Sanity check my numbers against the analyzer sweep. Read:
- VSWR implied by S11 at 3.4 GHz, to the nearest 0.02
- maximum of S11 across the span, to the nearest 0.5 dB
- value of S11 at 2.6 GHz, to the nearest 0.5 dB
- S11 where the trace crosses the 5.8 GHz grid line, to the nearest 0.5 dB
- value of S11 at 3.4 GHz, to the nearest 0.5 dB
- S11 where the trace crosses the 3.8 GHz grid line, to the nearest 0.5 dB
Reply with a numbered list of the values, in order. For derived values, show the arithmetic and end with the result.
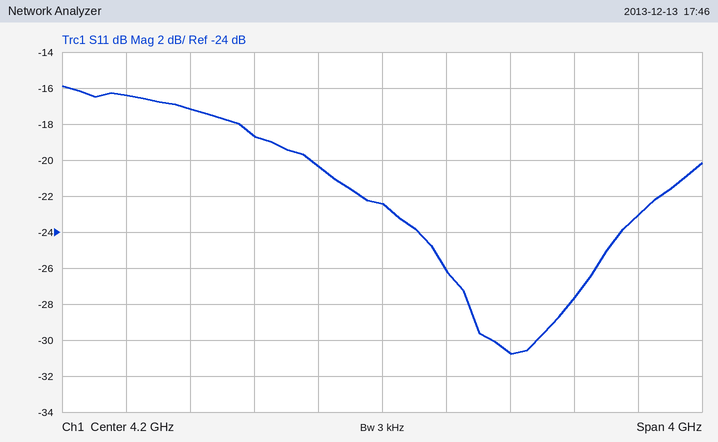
1. |Γ| = 10^(-18.5/20) = 0.1189; VSWR = (1 + 0.1189)/(1 − 0.1189) ≈ 1.27, so 1.26 to the nearest 0.02
2. -16.0 dB
3. -16.5 dB
4. -23.0 dB
5. -18.5 dB
6. -20.5 dB
